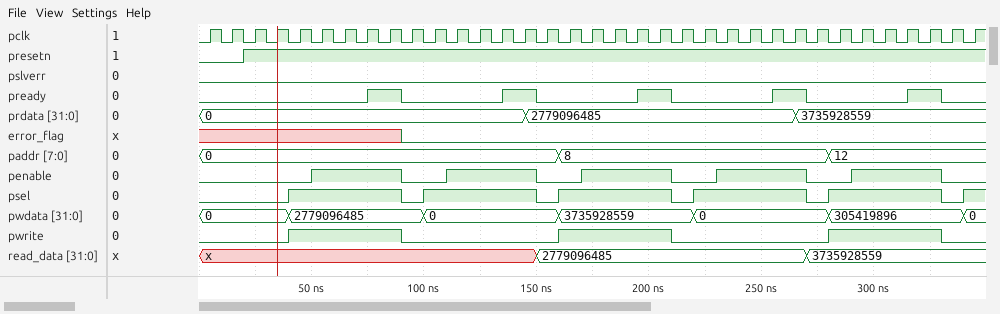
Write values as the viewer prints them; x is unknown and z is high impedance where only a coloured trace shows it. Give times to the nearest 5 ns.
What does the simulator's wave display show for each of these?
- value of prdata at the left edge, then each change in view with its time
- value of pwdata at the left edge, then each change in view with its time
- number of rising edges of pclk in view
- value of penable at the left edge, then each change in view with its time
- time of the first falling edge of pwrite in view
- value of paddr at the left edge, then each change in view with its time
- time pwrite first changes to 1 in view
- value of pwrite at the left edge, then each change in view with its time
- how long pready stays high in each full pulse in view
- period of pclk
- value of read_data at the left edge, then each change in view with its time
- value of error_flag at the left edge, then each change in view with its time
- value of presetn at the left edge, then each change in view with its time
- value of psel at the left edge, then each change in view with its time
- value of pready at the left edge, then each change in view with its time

0, 2779096485 at 145 ns, 3735928559 at 265 ns
0, 2779096485 at 40 ns, 0 at 100 ns, 3735928559 at 160 ns, 0 at 220 ns, 305419896 at 280 ns, 0 at 340 ns
35
0, 1 at 50 ns, 0 at 90 ns, 1 at 110 ns, 0 at 150 ns, 1 at 170 ns, 0 at 210 ns, 1 at 230 ns, 0 at 270 ns, 1 at 290 ns, 0 at 330 ns
90 ns
0, 8 at 160 ns, 12 at 280 ns
40 ns
0, 1 at 40 ns, 0 at 90 ns, 1 at 160 ns, 0 at 210 ns, 1 at 280 ns, 0 at 330 ns
15 ns, 15 ns, 15 ns, 15 ns, 15 ns
10 ns
x, 2779096485 at 150 ns, 3735928559 at 270 ns
x, 0 at 90 ns
0, 1 at 20 ns
0, 1 at 40 ns, 0 at 90 ns, 1 at 100 ns, 0 at 150 ns, 1 at 160 ns, 0 at 210 ns, 1 at 220 ns, 0 at 270 ns, 1 at 280 ns, 0 at 330 ns, 1 at 340 ns
0, 1 at 75 ns, 0 at 90 ns, 1 at 135 ns, 0 at 150 ns, 1 at 195 ns, 0 at 210 ns, 1 at 255 ns, 0 at 270 ns, 1 at 315 ns, 0 at 330 ns
